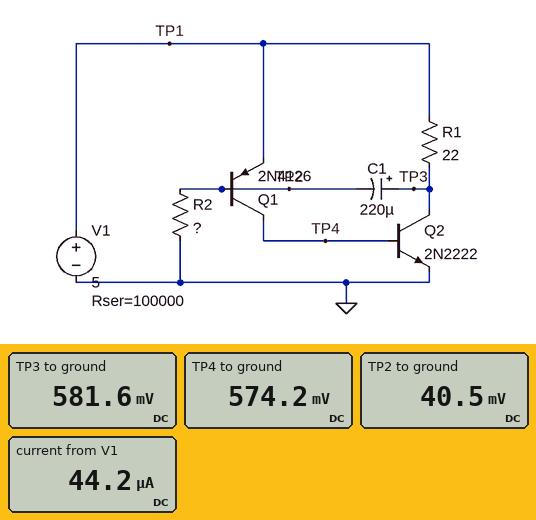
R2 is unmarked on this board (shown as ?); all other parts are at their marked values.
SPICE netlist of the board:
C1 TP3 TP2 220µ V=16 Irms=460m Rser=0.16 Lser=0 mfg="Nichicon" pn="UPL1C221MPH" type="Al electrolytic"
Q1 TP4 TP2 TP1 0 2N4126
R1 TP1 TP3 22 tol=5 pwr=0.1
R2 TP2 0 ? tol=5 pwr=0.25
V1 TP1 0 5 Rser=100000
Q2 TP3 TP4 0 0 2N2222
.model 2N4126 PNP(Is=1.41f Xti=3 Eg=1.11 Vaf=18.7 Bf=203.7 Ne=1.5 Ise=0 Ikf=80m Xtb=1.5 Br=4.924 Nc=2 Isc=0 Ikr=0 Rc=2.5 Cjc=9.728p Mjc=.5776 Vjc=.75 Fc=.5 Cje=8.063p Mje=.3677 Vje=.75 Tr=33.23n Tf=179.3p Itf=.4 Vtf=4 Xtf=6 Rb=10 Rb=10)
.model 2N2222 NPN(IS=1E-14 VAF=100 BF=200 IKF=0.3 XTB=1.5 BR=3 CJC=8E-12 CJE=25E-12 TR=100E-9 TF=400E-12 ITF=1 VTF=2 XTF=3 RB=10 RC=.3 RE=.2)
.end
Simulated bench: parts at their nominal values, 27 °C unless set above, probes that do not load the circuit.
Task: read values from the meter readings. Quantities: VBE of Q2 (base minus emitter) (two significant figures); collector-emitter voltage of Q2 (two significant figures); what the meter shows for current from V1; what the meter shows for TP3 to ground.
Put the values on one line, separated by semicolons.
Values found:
570 mV; 580 mV; 44.2 µA; 581.6 mV
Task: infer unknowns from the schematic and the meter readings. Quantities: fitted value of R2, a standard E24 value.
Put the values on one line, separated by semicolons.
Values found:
150 kΩ
